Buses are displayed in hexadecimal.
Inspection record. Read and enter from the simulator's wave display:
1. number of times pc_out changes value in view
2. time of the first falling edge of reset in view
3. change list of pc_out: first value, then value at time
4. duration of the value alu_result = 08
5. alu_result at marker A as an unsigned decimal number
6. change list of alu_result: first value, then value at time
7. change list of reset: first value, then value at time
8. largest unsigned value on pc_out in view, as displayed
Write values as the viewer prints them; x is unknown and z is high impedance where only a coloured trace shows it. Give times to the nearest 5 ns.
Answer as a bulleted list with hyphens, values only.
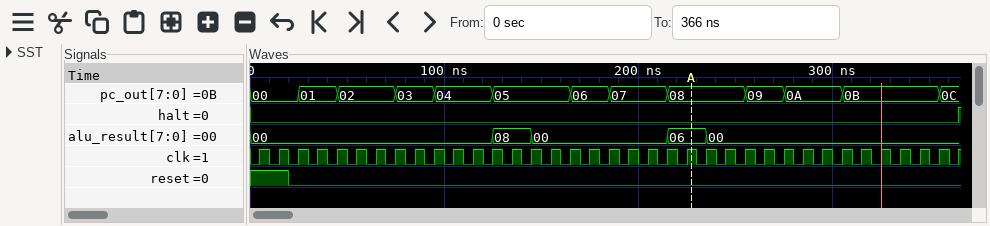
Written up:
- 12
- 20 ns
- 00, 01 at 25 ns, 02 at 45 ns, 03 at 75 ns, 04 at 95 ns, 05 at 125 ns, 06 at 165 ns, 07 at 185 ns, 08 at 215 ns, 09 at 255 ns, 0A at 275 ns, 0B at 305 ns, 0C at 355 ns
- 20 ns
- 6
- 00, 08 at 125 ns, 00 at 145 ns, 06 at 215 ns, 00 at 235 ns
- 1, 0 at 20 ns
- 0C
